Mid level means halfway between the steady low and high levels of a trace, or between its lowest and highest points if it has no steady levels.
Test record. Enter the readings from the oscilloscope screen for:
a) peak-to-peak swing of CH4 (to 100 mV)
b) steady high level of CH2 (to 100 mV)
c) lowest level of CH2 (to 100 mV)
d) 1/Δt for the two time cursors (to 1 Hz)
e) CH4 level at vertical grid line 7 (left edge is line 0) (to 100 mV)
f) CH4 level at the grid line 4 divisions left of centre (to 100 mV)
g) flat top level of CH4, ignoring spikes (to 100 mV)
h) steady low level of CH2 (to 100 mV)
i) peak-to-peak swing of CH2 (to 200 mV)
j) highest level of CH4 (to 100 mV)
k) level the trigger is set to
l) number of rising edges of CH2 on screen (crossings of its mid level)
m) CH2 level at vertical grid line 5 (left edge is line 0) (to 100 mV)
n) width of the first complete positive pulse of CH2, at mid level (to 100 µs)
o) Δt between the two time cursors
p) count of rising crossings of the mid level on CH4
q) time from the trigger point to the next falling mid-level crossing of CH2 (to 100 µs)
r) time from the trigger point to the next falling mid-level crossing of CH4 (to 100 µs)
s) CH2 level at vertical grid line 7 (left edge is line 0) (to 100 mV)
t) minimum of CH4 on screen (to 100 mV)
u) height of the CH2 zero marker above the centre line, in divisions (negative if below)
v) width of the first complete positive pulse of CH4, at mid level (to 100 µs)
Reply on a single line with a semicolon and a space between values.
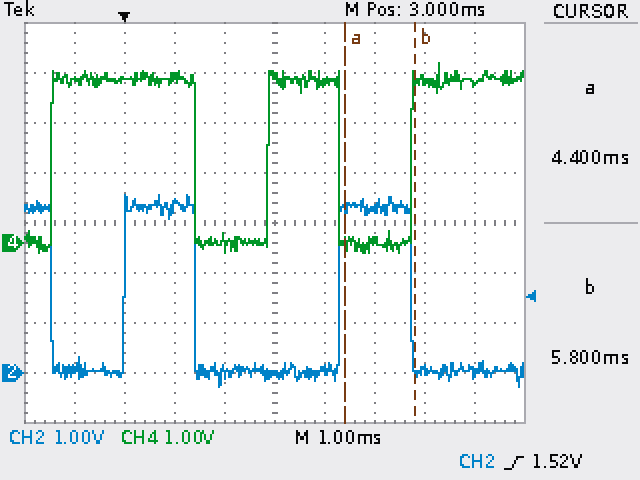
3.8 V; 3.3 V; -300 mV; 714 Hz; 0.0 V; 3.2 V; 3.3 V; 0.0 V; 3.8 V; 3.6 V; 1.52 V; 2; 0.0 V; 1.4 ms; 1.4 ms; 3; 1.4 ms; 1.4 ms; 3.3 V; -200 mV; -3.0 div; 2.9 ms
